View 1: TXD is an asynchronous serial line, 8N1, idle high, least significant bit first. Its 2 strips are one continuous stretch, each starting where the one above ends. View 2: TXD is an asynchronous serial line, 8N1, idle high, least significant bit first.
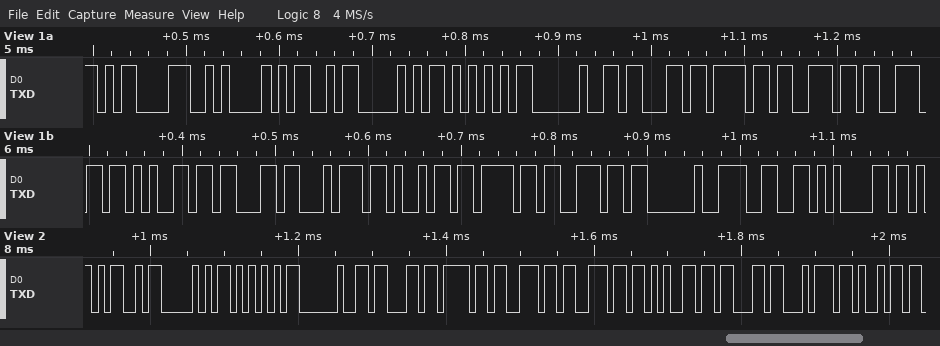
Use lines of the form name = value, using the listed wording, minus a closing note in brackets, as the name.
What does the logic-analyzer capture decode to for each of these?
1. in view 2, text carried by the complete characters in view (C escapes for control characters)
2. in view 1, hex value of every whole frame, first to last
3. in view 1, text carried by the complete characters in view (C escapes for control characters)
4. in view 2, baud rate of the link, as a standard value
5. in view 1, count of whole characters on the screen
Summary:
in view 2, text carried by the complete characters in view = "MPU connecti"
in view 1, hex value of every whole frame, first to last = 0x0D 0x0A 0x4D 0x50 0x55 0x20 0x63 0x6F 0x6E 0x6E 0x65 0x63 0x74 0x69 0x6F 0x6E 0x20 0x66 0x61
in view 1, text carried by the complete characters in view = "\r\nMPU connection fa"
in view 2, baud rate of the link, as a standard value = 115200 baud
in view 1, count of whole characters on the screen = 19
